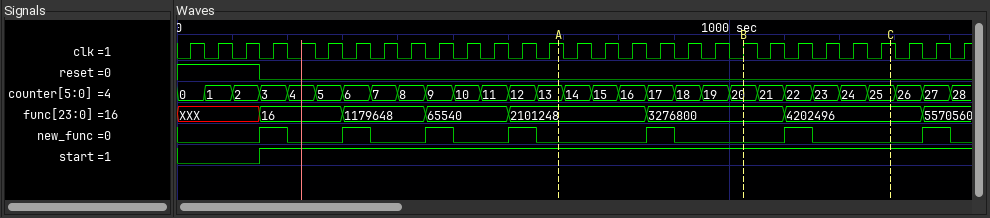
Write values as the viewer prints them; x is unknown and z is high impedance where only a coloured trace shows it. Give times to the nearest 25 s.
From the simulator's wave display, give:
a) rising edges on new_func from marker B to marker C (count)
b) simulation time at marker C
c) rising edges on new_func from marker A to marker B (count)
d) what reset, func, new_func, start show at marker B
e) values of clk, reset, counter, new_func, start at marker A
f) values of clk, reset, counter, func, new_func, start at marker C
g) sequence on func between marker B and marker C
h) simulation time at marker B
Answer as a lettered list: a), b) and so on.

a) 1
b) 1300 s
c) 1
d) reset=0, func=3276800, new_func=0, start=1
e) clk=1, reset=0, counter=13, new_func=0, start=1
f) clk=1, reset=0, counter=25, func=4202496, new_func=0, start=1
g) 3276800, 4202496
h) 1025 s
